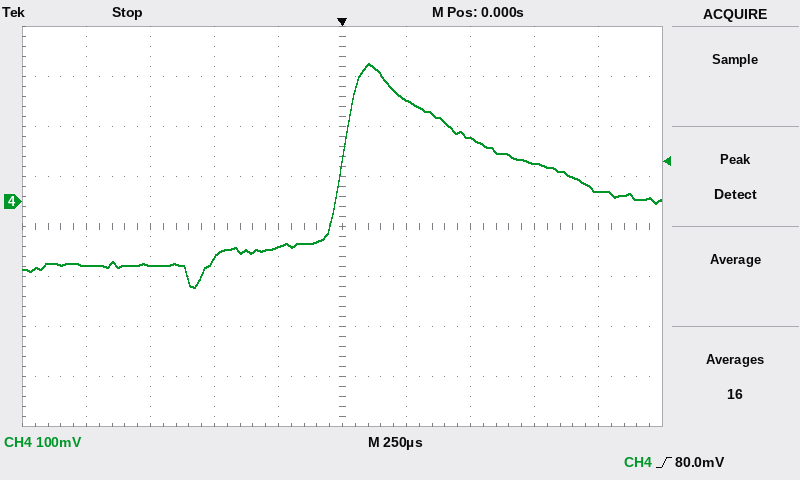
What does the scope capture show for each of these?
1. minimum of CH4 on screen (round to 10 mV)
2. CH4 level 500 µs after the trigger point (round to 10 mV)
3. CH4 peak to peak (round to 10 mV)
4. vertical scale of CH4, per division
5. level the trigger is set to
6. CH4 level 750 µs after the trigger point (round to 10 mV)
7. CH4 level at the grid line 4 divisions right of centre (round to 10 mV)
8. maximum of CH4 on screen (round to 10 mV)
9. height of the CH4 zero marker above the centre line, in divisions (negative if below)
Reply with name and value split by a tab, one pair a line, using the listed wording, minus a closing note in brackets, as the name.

minimum of CH4 on screen	-170 mV
CH4 level 500 µs after the trigger point	130 mV
CH4 peak to peak	450 mV
vertical scale of CH4, per division	100 mV
level the trigger is set to	80.0 mV
CH4 level 750 µs after the trigger point	80 mV
CH4 level at the grid line 4 divisions right of centre	20 mV
maximum of CH4 on screen	280 mV
height of the CH4 zero marker above the centre line, in divisions	+0.5 div
